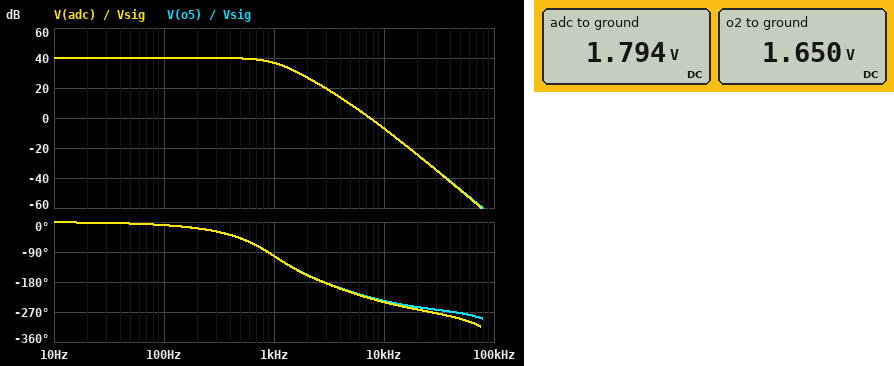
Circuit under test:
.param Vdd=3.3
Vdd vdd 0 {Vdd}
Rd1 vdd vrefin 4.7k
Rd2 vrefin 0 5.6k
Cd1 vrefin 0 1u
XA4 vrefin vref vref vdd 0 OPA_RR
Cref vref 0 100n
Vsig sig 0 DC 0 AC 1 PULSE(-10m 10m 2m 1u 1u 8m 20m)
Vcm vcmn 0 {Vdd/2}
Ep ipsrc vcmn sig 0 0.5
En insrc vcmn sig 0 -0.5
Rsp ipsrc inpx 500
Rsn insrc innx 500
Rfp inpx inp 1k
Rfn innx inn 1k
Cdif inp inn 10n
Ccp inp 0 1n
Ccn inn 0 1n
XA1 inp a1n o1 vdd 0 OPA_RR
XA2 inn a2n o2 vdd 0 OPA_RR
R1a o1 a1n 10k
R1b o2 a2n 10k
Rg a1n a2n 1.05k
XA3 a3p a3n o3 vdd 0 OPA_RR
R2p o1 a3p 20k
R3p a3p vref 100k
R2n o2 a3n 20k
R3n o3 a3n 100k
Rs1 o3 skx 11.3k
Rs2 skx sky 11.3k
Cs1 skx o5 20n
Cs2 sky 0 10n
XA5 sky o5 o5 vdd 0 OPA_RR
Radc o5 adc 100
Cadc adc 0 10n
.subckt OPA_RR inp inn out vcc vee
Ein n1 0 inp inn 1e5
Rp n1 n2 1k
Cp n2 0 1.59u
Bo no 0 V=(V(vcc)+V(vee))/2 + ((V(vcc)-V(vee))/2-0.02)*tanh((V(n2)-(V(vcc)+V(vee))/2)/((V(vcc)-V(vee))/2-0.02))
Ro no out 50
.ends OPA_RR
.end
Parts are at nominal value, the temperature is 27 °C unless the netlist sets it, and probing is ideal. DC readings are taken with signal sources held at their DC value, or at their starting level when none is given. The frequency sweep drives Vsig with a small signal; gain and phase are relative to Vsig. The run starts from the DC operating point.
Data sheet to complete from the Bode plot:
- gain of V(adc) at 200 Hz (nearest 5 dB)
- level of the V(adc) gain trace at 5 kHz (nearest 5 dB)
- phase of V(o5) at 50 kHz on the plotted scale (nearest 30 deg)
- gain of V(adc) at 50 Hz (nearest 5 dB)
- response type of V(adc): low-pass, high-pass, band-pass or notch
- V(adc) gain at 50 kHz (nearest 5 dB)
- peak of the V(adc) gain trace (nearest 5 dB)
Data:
40 dB
10 dB
-270 deg
40 dB
low-pass
-50 dB
40 dB
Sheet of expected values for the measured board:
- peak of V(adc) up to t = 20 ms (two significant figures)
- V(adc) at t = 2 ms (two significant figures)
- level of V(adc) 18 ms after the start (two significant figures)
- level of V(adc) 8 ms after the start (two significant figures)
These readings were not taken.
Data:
2.9 V
790 mV
790 mV
2.8 V
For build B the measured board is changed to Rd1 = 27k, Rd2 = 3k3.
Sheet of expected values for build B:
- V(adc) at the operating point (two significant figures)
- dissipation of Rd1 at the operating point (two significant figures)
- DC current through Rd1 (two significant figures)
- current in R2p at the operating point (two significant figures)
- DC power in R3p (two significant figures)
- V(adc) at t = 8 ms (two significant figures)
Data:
360 mV
320 µW
110 µA
11 µA
12 µW
1.4 V
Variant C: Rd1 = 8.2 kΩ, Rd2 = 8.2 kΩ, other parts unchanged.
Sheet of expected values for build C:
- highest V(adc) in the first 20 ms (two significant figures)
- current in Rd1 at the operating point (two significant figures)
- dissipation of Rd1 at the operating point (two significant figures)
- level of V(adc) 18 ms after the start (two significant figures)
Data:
2.7 V
200 µA
330 µW
650 mV
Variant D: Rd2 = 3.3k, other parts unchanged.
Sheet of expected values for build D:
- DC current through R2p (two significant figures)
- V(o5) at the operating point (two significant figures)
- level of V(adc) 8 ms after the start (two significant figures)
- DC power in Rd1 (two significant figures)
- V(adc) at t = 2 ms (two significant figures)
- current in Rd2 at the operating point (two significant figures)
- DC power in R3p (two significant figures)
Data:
2.4 µA
1.4 V
2.4 V
800 µW
360 mV
410 µA
580 nW
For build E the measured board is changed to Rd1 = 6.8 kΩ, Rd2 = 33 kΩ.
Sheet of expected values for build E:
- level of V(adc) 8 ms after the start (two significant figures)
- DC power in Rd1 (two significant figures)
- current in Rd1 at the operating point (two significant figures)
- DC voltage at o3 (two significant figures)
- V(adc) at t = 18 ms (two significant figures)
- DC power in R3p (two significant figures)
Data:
3.3 V
47 µW
83 µA
2.7 V
1.7 V
8.2 µW
